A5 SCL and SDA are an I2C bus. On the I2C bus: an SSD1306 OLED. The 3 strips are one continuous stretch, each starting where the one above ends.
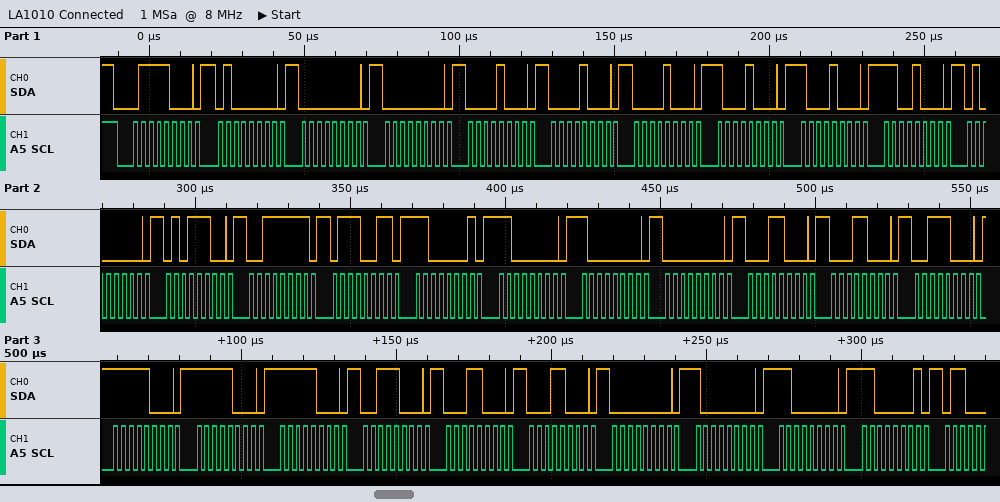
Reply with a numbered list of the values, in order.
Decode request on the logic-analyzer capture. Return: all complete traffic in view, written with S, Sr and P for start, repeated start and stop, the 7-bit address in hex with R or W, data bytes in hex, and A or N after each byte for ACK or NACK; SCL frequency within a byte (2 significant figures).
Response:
1. S 3CW A 40 A 00 A 00 A 08 A 08 A 08 A 88 A 88 A C8 A 40 A 5C A 3F A 73 A C1 A C0 A 80 A 00 A 18 A 18 A 38 A F8 A F8 A F8 A 38 A 18 A 18 A 00 A 80 A C0 A C1 A
2. 400 kHz
